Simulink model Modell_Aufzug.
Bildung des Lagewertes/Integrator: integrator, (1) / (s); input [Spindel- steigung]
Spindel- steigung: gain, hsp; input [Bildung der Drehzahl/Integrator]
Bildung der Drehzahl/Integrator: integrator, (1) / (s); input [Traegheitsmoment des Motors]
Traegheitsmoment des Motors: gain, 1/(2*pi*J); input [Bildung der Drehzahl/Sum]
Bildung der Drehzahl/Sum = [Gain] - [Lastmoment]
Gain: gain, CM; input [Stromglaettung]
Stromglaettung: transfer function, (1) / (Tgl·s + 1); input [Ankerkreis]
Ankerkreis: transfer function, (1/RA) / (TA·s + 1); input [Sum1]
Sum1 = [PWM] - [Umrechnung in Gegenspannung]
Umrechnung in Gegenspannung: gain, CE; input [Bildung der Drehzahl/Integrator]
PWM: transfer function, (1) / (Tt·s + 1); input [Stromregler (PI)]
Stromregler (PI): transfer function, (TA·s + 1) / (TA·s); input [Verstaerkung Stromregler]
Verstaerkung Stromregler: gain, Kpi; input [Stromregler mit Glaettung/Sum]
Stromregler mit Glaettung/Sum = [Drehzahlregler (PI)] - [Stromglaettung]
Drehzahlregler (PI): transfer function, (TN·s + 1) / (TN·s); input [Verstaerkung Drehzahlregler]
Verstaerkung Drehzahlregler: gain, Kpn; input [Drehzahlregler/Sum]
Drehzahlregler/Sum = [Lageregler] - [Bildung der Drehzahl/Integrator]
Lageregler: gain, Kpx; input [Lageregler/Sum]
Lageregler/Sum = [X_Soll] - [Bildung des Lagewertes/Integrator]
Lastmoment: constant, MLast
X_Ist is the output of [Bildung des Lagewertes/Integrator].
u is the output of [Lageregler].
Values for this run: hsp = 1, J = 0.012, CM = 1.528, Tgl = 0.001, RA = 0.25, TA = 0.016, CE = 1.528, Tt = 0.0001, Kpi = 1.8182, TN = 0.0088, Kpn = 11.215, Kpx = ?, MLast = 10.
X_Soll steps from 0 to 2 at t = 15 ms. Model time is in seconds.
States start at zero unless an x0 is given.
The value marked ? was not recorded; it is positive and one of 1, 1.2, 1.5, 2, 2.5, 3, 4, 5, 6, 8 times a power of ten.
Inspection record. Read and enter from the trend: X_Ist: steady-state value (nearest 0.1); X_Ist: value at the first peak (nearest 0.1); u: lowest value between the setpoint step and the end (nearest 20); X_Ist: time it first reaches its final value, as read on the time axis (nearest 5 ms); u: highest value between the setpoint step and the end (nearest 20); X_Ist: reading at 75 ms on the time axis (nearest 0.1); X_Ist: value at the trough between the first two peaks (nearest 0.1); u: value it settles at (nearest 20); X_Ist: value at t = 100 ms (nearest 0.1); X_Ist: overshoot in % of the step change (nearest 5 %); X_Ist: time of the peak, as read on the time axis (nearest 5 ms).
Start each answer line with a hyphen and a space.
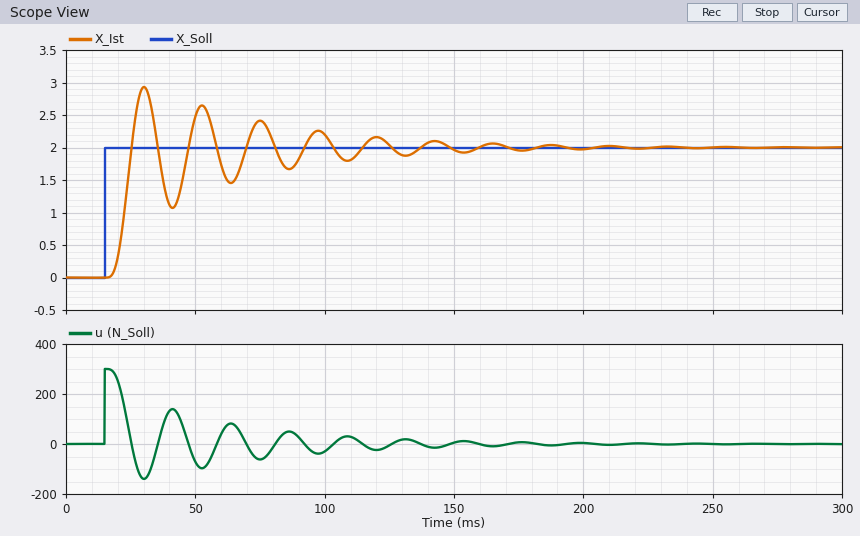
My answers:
- 2.0
- 2.9
- -140
- 25 ms
- 300
- 2.4
- 1.1
- 0
- 2.2
- 45 %
- 30 ms
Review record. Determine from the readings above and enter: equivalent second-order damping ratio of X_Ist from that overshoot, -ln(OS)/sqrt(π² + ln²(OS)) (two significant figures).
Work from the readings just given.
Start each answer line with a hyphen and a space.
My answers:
- 0.25
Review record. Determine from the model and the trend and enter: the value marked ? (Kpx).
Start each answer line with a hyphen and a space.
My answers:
- 150
